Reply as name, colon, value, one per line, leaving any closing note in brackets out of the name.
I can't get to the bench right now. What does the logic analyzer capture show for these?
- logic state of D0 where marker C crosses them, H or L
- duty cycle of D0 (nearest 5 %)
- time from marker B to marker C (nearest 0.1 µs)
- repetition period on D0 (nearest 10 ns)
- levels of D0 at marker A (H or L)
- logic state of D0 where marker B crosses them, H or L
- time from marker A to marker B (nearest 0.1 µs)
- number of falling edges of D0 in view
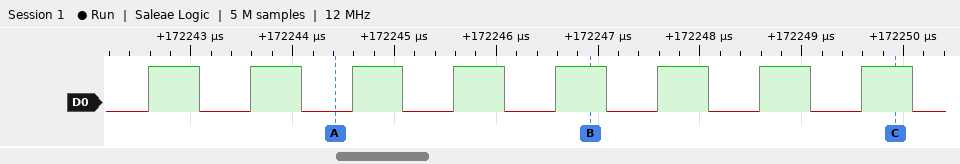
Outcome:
logic state of D0 where marker C crosses them, H or L: D0=H
duty cycle of D0: 50 %
time from marker B to marker C: 3 µs
repetition period on D0: 1000 ns
levels of D0 at marker A: D0=L
logic state of D0 where marker B crosses them, H or L: D0=H
time from marker A to marker B: 2.5 µs
number of falling edges of D0 in view: 8
